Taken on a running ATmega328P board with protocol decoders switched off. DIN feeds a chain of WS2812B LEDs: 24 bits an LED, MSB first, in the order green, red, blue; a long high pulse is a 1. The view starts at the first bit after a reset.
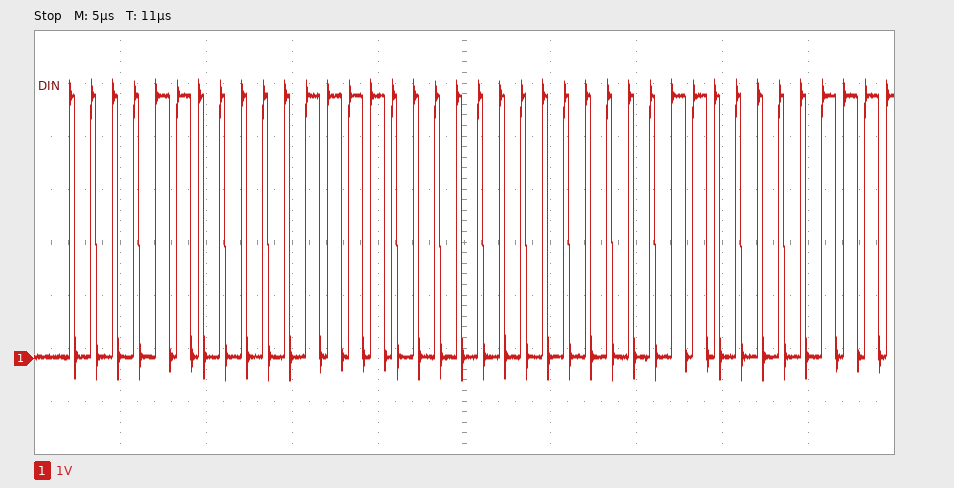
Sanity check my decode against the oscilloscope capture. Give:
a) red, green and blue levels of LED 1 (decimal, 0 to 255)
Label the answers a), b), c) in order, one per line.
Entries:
a) 30, 12, 0
